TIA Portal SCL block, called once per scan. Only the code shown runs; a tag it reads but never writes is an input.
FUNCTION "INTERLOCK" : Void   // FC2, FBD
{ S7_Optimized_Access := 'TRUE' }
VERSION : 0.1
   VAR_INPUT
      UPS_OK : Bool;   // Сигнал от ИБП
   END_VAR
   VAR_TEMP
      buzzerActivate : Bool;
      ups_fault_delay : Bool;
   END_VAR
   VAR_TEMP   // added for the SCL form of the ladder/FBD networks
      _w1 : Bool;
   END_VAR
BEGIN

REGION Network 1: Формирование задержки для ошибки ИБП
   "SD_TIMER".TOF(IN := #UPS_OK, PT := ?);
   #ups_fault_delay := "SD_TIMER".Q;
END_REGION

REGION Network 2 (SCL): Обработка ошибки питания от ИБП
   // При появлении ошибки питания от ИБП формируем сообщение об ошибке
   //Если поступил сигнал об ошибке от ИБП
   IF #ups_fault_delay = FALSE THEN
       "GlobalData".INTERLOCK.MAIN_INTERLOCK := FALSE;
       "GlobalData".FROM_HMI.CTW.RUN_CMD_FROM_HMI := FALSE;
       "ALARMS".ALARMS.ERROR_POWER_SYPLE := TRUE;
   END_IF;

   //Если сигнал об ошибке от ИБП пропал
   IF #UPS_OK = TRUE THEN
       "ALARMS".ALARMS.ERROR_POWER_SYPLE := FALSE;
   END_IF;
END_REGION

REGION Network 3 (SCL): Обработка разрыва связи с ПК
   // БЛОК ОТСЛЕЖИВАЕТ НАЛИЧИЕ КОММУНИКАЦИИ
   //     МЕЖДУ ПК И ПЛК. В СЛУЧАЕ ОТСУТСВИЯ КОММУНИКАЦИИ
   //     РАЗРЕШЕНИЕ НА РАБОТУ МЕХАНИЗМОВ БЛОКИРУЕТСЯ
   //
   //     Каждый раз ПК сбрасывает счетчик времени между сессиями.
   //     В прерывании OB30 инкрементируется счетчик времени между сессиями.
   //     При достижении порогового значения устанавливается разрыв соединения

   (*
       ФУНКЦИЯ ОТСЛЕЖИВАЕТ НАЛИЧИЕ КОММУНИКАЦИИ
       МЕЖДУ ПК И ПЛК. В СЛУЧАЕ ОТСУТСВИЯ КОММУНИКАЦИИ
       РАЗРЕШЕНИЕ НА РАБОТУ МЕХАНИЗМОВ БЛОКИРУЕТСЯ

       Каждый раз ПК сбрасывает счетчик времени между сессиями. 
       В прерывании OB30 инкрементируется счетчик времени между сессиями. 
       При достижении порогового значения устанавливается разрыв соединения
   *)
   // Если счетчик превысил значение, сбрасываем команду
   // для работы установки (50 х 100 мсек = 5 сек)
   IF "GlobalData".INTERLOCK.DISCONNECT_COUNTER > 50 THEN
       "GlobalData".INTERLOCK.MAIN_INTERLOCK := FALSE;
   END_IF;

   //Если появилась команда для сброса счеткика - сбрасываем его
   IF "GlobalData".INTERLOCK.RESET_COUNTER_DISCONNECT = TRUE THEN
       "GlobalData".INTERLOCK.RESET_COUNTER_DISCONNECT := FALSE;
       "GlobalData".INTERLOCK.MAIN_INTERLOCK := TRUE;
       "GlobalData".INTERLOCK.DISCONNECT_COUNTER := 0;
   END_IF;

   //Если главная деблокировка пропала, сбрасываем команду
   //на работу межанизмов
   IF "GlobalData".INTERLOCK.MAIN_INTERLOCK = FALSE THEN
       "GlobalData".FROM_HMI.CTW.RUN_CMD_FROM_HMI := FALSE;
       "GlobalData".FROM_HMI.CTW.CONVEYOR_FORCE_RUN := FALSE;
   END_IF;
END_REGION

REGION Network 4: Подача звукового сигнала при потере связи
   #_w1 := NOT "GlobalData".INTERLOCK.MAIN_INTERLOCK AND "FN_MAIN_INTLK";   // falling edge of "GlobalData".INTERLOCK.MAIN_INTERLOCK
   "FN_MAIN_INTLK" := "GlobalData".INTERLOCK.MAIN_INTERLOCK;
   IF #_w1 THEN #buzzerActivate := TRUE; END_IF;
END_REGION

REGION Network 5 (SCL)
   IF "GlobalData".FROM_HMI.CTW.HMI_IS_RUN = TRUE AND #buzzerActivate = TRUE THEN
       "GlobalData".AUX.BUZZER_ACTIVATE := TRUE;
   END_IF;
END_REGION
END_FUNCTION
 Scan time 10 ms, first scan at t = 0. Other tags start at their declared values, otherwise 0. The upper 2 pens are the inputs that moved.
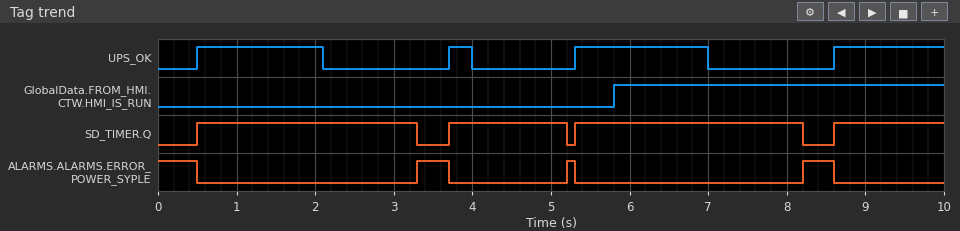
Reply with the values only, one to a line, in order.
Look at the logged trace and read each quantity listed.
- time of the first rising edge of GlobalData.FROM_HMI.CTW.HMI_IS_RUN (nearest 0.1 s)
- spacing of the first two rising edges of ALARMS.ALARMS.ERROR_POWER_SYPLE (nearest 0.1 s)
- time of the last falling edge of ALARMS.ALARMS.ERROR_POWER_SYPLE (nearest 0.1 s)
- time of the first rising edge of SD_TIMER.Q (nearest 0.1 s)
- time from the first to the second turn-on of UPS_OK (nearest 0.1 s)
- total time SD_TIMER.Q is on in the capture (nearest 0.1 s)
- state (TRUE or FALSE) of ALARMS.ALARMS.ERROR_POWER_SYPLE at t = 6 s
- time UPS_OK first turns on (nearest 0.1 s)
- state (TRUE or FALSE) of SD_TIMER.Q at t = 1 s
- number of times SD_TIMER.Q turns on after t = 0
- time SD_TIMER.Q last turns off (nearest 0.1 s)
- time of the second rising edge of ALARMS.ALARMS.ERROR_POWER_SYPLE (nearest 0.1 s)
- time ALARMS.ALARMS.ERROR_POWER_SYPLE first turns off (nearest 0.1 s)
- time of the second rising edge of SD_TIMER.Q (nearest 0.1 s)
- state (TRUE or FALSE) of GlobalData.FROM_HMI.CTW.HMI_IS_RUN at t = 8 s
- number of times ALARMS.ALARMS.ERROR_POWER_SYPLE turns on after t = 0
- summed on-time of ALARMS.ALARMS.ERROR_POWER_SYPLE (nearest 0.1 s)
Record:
5.8 s
1.9 s
8.6 s
0.5 s
3.2 s
8.6 s
FALSE
0.5 s
TRUE
4
8.2 s
5.2 s
0.5 s
3.7 s
TRUE
3
1.4 s
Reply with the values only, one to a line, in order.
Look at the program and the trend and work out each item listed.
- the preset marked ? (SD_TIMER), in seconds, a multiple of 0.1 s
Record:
1.2 s
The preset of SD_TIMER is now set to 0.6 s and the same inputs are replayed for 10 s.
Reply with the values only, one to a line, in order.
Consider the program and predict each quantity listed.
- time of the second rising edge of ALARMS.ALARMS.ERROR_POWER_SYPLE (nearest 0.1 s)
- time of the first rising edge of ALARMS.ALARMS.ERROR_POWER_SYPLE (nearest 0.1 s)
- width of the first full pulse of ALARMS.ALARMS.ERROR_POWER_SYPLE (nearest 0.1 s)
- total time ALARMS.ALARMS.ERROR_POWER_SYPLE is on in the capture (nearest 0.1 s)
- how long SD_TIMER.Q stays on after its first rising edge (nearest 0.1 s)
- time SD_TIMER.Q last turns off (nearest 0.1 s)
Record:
4.6 s
2.7 s
1.0 s
3.2 s
2.2 s
7.6 s
